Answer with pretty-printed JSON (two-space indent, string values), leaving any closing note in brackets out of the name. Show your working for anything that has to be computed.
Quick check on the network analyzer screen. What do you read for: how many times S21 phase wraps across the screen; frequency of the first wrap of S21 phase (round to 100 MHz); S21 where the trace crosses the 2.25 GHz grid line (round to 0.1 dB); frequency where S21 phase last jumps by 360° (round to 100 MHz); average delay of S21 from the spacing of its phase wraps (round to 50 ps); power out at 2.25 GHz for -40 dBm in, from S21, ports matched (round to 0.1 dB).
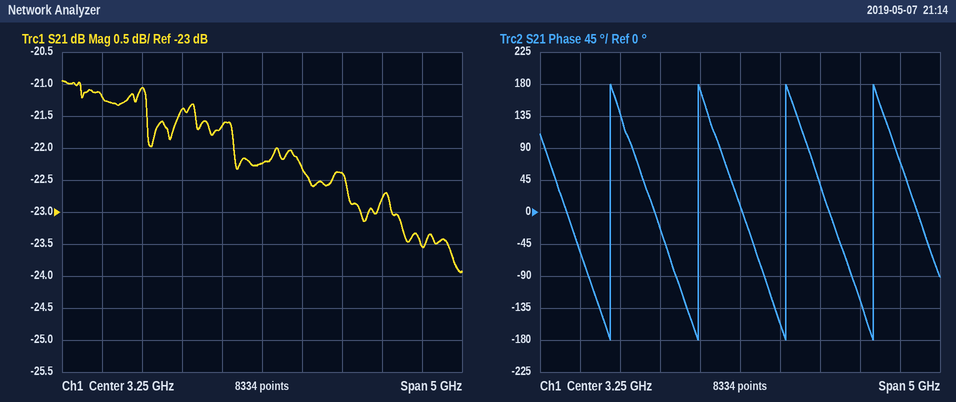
{
  "how many times S21 phase wraps across the screen": "4",
  "frequency of the first wrap of S21 phase": "1.6 GHz",
  "S21 where the trace crosses the 2.25 GHz grid line": "-21.4 dB",
  "frequency where S21 phase last jumps by 360°": "4.9 GHz",
  "average delay of S21 from the spacing of its phase wraps": "3 cycles / (4.9 GHz − 1.6 GHz) ≈ 909 ps, so 900 ps to the nearest 50 ps",
  "power out at 2.25 GHz for -40 dBm in, from S21, ports matched": "-40 dBm + (-21.4 dB) = -61.4 dBm"
}
